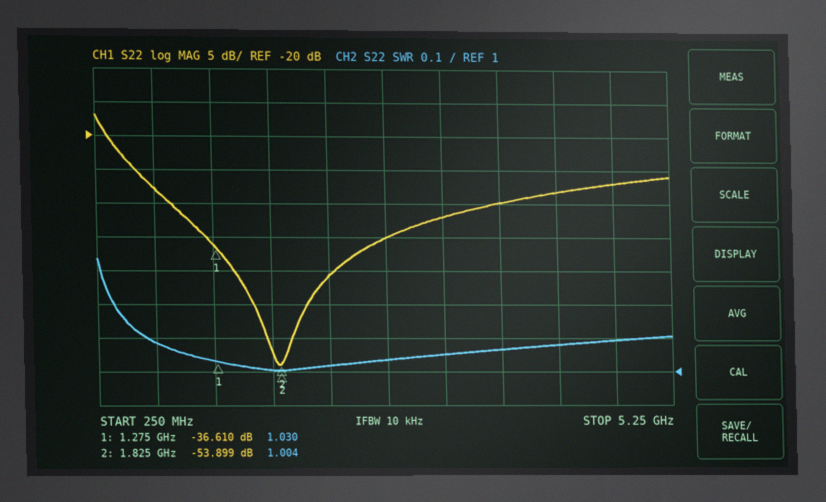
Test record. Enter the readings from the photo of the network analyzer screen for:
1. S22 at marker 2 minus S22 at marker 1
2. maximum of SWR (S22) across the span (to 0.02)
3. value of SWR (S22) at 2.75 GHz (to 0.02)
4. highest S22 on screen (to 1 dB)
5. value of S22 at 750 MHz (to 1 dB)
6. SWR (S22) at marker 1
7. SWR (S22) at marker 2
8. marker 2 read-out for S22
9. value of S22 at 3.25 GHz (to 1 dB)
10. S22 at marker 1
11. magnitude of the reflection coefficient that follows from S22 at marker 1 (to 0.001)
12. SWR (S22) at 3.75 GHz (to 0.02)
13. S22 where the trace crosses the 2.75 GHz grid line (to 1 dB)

-17.289 dB
1.34
1.04
-17 dB
-28 dB
1.030
1.004
-53.899 dB
-32 dB
-36.610 dB
0.015
1.06
-35 dB
